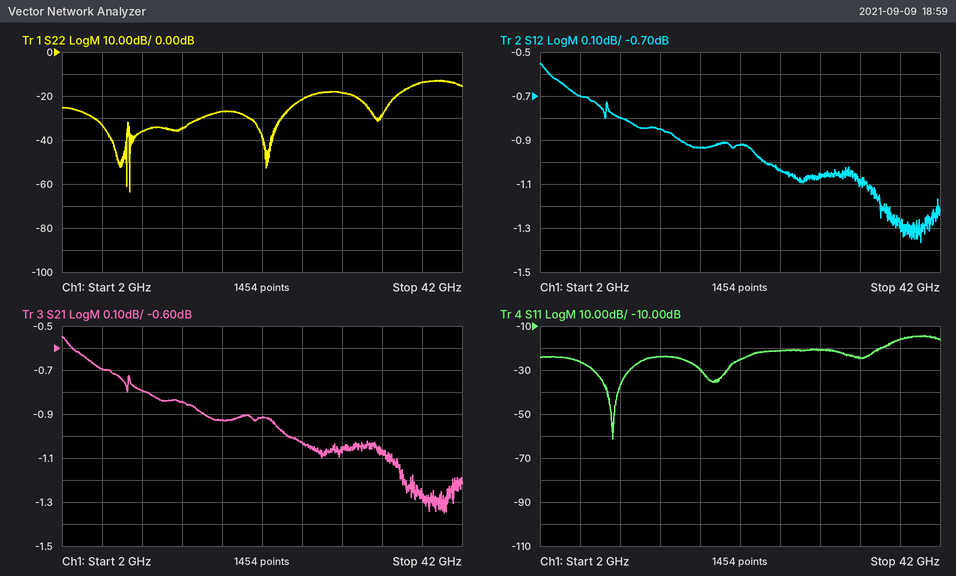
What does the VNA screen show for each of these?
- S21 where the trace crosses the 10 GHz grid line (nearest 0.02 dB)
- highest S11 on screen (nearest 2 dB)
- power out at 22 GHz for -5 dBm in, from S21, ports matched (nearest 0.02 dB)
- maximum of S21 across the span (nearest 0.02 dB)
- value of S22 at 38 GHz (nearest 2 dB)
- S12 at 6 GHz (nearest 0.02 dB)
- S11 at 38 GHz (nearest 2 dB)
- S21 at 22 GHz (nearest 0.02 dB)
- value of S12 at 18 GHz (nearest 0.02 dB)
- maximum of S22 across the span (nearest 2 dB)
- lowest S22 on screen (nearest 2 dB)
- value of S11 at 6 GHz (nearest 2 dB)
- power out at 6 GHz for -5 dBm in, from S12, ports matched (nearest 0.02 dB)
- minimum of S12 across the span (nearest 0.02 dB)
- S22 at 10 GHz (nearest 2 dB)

-0.80 dB
-14 dB
-5.92 dBm
-0.54 dB
-14 dB
-0.70 dB
-16 dB
-0.92 dB
-0.94 dB
-12 dB
-64 dB
-26 dB
-5.70 dBm
-1.36 dB
-36 dB
